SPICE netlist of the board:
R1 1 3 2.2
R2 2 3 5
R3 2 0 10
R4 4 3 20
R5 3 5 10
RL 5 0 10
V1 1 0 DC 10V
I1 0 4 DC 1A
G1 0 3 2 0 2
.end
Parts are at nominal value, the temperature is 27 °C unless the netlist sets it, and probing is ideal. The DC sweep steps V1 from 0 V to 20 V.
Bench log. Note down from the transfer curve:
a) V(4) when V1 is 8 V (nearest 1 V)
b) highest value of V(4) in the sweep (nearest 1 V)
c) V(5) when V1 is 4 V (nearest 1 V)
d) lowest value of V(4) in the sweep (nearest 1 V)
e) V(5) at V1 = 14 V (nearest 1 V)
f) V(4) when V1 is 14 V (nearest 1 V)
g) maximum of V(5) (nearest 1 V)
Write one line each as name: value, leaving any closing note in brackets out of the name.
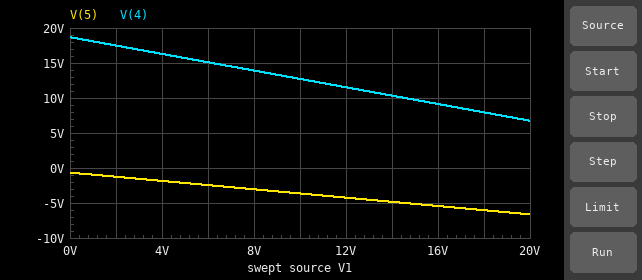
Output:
V(4) when V1 is 8 V: 14 V
highest value of V(4) in the sweep: 19 V
V(5) when V1 is 4 V: -2 V
lowest value of V(4) in the sweep: 7 V
V(5) at V1 = 14 V: -5 V
V(4) when V1 is 14 V: 10 V
maximum of V(5): -1 V
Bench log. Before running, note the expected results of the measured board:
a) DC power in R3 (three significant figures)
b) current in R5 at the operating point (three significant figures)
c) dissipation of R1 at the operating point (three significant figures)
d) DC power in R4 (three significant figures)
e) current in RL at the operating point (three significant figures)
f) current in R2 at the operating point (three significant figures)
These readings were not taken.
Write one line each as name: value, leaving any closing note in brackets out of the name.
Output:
DC power in R3: 2.35 W
current in R5 at the operating point: 364 mA
dissipation of R1 at the operating point: 136 W
DC power in R4: 20.0 W
current in RL at the operating point: 364 mA
current in R2 at the operating point: 485 mA
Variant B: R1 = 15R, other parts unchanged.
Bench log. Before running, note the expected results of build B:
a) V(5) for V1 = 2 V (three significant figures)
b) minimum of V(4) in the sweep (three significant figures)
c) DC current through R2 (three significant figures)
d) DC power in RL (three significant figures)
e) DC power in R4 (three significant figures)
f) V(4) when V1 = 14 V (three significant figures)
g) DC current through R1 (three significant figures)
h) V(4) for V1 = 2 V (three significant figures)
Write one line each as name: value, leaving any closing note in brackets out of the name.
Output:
V(5) for V1 = 2 V: -493 mV
minimum of V(4) in the sweep: 18.0 V
DC current through R2: 96.6 mA
DC power in RL: 52.5 mW
DC power in R4: 20.0 W
V(4) when V1 = 14 V: 18.3 V
DC current through R1: 763 mA
V(4) for V1 = 2 V: 19.0 V
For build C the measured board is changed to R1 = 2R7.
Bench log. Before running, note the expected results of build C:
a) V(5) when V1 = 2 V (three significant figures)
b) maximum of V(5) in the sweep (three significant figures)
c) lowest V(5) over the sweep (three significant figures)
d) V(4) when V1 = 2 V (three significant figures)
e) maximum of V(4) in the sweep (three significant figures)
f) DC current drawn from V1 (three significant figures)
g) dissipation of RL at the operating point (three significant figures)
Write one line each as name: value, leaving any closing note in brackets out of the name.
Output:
V(5) when V1 = 2 V: -1.03 V
maximum of V(5) in the sweep: -591 mV
lowest V(5) over the sweep: -4.97 V
V(4) when V1 = 2 V: 17.9 V
maximum of V(4) in the sweep: 18.8 V
DC current drawn from V1: 5.76 A
dissipation of RL at the operating point: 772 mW
